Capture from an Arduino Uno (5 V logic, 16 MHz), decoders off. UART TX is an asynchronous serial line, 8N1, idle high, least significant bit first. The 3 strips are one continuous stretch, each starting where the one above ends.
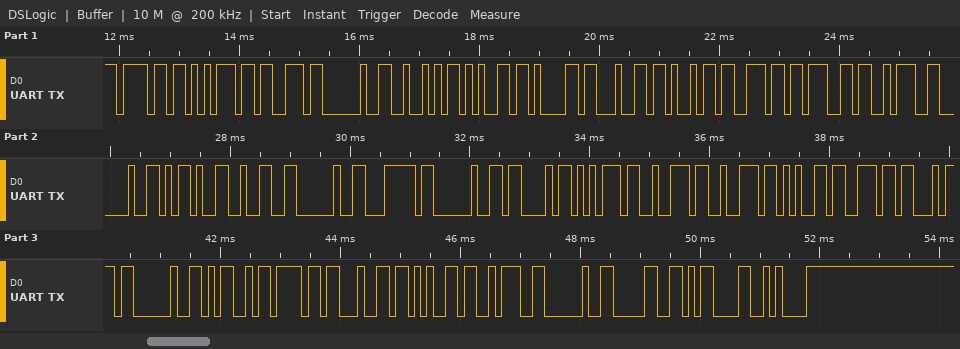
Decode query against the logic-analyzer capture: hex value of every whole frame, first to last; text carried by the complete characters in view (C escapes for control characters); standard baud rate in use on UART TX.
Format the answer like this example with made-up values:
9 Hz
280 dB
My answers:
6F 75 73 20 52 65 61 64 69 6E 67 3A 20 2D 32 20 7C 20 43 75 72 72 65 6E 74 20 4D 6F 64 65 3A 20 30 0D 0A
"ous Reading: -2 | Current Mode: 0\r\n"
9600 baud
